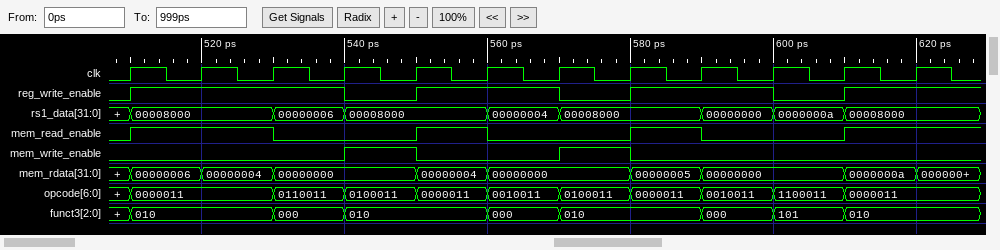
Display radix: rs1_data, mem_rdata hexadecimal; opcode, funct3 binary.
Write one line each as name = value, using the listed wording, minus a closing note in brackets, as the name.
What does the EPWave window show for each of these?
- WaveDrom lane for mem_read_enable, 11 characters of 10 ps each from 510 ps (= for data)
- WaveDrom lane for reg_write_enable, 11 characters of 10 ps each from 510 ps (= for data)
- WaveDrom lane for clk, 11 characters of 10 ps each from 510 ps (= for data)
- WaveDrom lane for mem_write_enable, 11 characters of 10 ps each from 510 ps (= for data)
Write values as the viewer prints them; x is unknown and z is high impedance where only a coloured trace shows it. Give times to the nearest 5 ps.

WaveDrom lane for mem_read_enable, 11 characters of 10 ps each from 510 ps = {name: 'mem_read_enable', wave: '1.0.10.10.1'}
WaveDrom lane for reg_write_enable, 11 characters of 10 ps each from 510 ps = {name: 'reg_write_enable', wave: '1..01.01.01'}
WaveDrom lane for clk, 11 characters of 10 ps each from 510 ps = {name: 'clk', wave: 'p..........'}
WaveDrom lane for mem_write_enable, 11 characters of 10 ps each from 510 ps = {name: 'mem_write_enable', wave: '0..10.10...'}
